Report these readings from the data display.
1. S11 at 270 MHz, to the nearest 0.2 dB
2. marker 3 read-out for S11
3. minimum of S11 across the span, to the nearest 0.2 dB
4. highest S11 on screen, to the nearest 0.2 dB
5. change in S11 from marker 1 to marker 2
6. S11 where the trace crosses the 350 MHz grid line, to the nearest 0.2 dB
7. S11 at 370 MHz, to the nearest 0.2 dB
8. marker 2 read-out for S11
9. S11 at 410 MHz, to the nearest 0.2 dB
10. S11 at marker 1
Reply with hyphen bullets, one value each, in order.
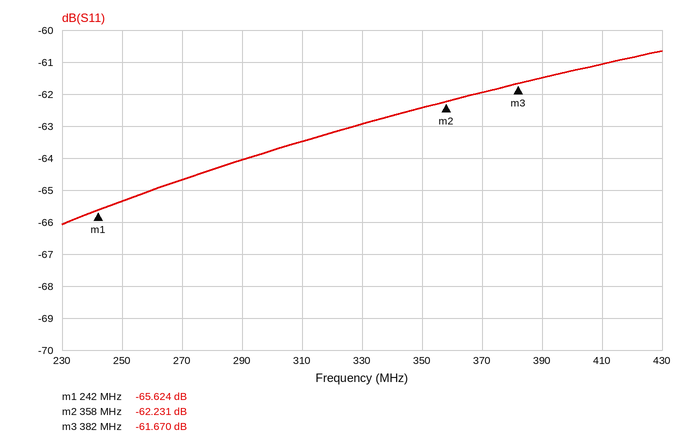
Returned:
- -64.6 dB
- -61.670 dB
- -66.0 dB
- -60.6 dB
- 3.393 dB
- -62.4 dB
- -62.0 dB
- -62.231 dB
- -61.0 dB
- -65.624 dB
